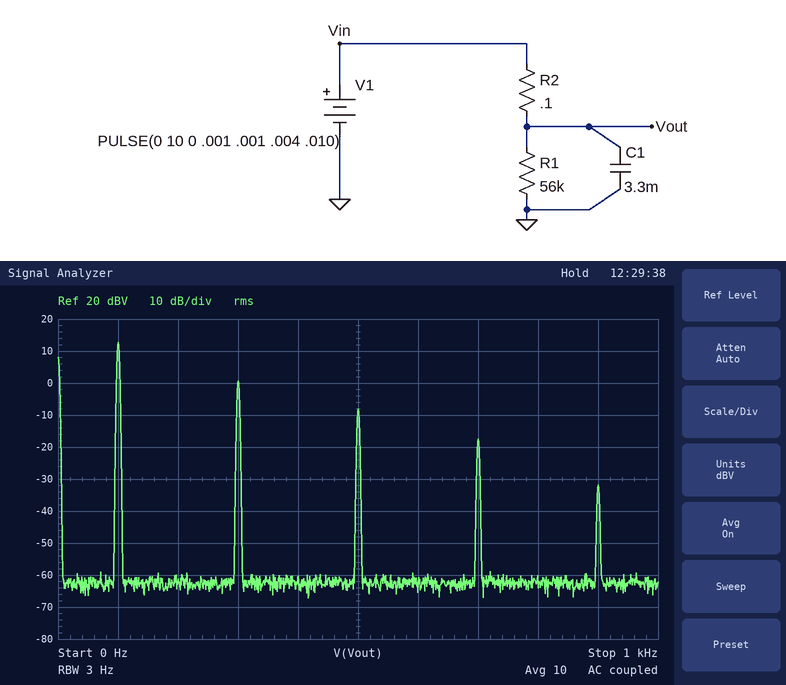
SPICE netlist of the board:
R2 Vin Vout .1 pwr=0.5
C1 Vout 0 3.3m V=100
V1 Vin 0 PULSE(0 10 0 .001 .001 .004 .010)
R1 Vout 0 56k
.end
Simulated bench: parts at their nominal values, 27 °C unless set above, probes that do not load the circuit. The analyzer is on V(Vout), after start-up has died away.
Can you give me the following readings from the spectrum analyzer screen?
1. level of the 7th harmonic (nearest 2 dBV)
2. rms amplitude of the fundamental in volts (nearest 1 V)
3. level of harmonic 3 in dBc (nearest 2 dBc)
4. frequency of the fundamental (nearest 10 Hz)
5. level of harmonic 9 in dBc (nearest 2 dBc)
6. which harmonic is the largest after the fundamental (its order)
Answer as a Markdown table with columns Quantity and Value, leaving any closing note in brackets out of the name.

| Quantity | Value |
|---|---|
| level of the 7th harmonic | -18 dBV |
| rms amplitude of the fundamental in volts | 4 V |
| level of harmonic 3 in dBc | -12 dBc |
| frequency of the fundamental | 100 Hz |
| level of harmonic 9 in dBc | -44 dBc |
| which harmonic is the largest after the fundamental | 3 |
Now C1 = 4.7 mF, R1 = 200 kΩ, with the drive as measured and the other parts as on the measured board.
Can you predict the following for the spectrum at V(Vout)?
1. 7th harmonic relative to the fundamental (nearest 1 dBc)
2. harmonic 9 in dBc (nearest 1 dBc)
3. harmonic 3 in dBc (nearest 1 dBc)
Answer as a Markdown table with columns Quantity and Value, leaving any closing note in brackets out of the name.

| Quantity | Value |
|---|---|
| 7th harmonic relative to the fundamental | -32 dBc |
| harmonic 9 in dBc | -47 dBc |
| harmonic 3 in dBc | -13 dBc |
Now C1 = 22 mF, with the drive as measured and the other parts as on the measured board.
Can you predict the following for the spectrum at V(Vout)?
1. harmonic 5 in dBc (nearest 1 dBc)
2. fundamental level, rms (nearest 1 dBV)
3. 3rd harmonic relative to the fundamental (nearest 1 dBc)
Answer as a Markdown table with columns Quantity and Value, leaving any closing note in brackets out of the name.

| Quantity | Value |
|---|---|
| harmonic 5 in dBc | -30 dBc |
| fundamental level, rms | 8 dBV |
| 3rd harmonic relative to the fundamental | -19 dBc |
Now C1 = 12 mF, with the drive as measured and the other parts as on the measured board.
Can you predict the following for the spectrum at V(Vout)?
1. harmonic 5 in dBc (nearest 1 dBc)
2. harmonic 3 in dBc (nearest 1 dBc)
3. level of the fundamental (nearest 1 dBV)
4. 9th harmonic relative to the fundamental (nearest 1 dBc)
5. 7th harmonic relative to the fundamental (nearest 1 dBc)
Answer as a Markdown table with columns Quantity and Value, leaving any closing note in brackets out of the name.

| Quantity | Value |
|---|---|
| harmonic 5 in dBc | -28 dBc |
| harmonic 3 in dBc | -17 dBc |
| level of the fundamental | 11 dBV |
| 9th harmonic relative to the fundamental | -53 dBc |
| 7th harmonic relative to the fundamental | -38 dBc |
